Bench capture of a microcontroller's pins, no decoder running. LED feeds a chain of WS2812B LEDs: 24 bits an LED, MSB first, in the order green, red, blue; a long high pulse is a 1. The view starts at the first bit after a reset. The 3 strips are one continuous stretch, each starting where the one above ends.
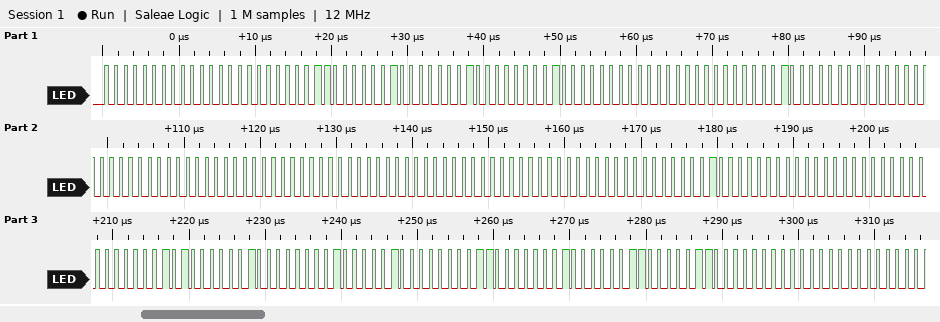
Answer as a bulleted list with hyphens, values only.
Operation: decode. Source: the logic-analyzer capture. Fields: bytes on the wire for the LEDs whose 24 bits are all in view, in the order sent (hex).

- 00 00 03 02 02 01 00 00 01 00 00 00 00 00 00 00 00 00 01 00 00 00 05 02 01 04 03 01 03 06
